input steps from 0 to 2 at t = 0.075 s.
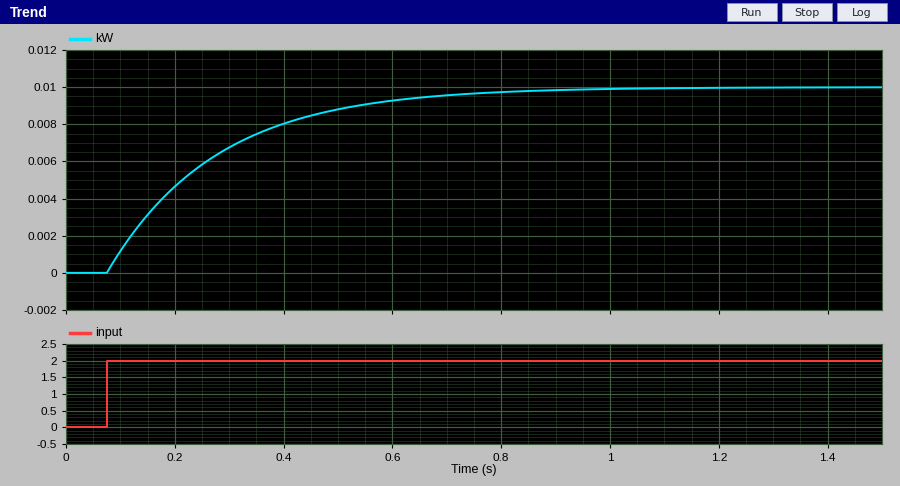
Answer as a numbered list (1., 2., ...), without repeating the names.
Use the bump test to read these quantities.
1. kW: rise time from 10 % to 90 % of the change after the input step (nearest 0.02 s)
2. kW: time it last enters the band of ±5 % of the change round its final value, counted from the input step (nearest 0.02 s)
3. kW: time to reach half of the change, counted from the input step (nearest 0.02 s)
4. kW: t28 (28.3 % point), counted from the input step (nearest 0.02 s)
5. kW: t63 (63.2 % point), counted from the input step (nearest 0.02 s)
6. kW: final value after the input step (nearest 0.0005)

1. 0.44 s
2. 0.60 s
3. 0.14 s
4. 0.06 s
5. 0.20 s
6. 0.0100
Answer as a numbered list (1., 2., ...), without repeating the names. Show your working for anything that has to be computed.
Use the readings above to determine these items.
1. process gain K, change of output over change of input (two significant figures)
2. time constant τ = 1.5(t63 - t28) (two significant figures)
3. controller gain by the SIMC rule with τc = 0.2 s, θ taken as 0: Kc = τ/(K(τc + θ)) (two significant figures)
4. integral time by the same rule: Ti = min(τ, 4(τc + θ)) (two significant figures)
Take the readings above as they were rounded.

1. (0.01 - 0) / 2 = 0.0050
2. 1.5 × (0.2 - 0.06) = 0.21 s
3. 0.21 / (0.005 × (0.2 + 0)) = 210
4. min(0.21, 4 × (0.2 + 0)) = 0.21 s
